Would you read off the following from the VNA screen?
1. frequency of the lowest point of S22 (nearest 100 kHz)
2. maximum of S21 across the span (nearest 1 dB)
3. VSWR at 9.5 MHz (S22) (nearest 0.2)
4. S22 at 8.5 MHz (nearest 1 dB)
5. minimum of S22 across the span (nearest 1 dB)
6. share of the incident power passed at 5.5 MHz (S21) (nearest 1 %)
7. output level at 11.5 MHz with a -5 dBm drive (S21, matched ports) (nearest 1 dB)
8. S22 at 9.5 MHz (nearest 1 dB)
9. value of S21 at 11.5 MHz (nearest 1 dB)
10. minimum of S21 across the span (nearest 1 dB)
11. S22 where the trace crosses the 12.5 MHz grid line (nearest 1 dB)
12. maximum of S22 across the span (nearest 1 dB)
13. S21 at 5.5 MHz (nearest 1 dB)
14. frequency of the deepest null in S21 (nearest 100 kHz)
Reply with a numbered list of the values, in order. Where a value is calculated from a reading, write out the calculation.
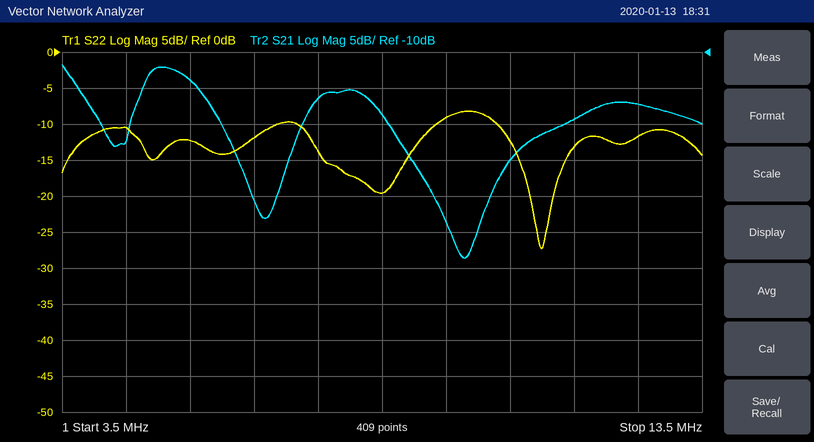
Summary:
1. 11.0 MHz
2. -12 dB
3. |Γ| = 10^(-9/20) = 0.3548; VSWR = (1 + 0.3548)/(1 − 0.3548) ≈ 2.10, so 2.0 to the nearest 0.2
4. -20 dB
5. -27 dB
6. 10^(-14/10) ≈ 4 %
7. -5 dBm + (-19 dB) = -24 dBm
8. -9 dB
9. -19 dB
10. -39 dB
11. -12 dB
12. -8 dB
13. -14 dB
14. 9.8 MHz
